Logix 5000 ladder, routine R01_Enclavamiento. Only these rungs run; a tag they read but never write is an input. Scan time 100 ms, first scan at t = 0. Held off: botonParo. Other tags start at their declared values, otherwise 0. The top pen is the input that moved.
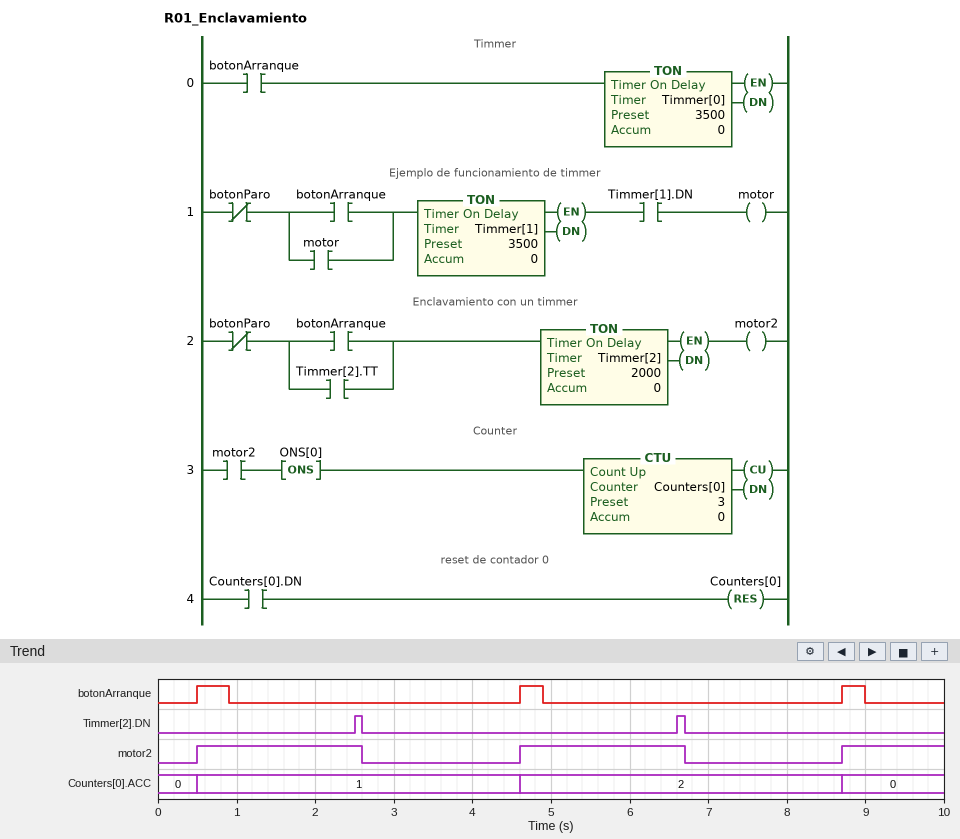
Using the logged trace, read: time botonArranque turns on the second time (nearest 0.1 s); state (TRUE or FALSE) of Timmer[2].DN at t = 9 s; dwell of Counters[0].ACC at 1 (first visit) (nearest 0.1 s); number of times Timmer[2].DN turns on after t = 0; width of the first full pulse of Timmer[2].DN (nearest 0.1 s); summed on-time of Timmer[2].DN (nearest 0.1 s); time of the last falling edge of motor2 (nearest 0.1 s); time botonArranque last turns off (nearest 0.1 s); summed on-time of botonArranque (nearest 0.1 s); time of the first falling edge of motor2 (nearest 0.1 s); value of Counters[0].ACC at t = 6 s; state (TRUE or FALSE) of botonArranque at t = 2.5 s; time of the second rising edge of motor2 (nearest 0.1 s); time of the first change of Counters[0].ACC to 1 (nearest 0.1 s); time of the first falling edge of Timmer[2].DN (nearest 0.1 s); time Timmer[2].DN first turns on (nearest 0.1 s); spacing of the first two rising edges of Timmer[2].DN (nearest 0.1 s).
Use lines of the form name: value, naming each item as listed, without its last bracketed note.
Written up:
time botonArranque turns on the second time: 4.6 s
state (TRUE or FALSE) of Timmer[2].DN at t = 9 s: FALSE
dwell of Counters[0].ACC at 1 (first visit): 4.1 s
number of times Timmer[2].DN turns on after t = 0: 2
width of the first full pulse of Timmer[2].DN: 0.1 s
summed on-time of Timmer[2].DN: 0.2 s
time of the last falling edge of motor2: 6.7 s
time botonArranque last turns off: 9.0 s
summed on-time of botonArranque: 1.0 s
time of the first falling edge of motor2: 2.6 s
value of Counters[0].ACC at t = 6 s: 2
state (TRUE or FALSE) of botonArranque at t = 2.5 s: FALSE
time of the second rising edge of motor2: 4.6 s
time of the first change of Counters[0].ACC to 1: 0.5 s
time of the first falling edge of Timmer[2].DN: 2.6 s
time Timmer[2].DN first turns on: 2.5 s
spacing of the first two rising edges of Timmer[2].DN: 4.1 s
